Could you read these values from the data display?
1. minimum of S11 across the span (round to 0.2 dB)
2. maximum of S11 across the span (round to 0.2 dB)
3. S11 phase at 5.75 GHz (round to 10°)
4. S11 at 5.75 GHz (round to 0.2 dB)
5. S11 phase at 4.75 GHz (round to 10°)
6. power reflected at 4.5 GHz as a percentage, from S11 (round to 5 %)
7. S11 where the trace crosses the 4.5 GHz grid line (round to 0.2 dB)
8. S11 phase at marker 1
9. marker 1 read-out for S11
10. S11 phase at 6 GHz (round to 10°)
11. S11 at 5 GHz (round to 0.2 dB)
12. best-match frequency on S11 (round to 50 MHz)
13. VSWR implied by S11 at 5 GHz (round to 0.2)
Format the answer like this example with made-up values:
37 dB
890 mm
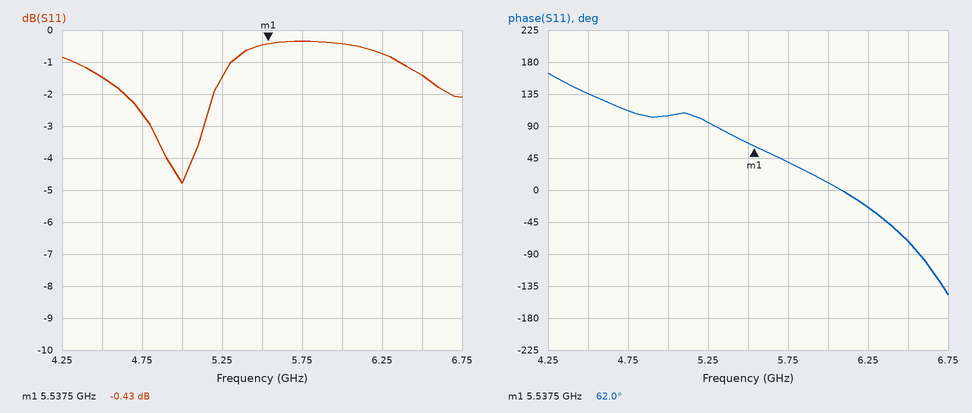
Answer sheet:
-4.8 dB
-0.4 dB
40°
-0.4 dB
110°
70 %
-1.4 dB
62.0°
-0.43 dB
10°
-4.8 dB
5.00 GHz
3.8
